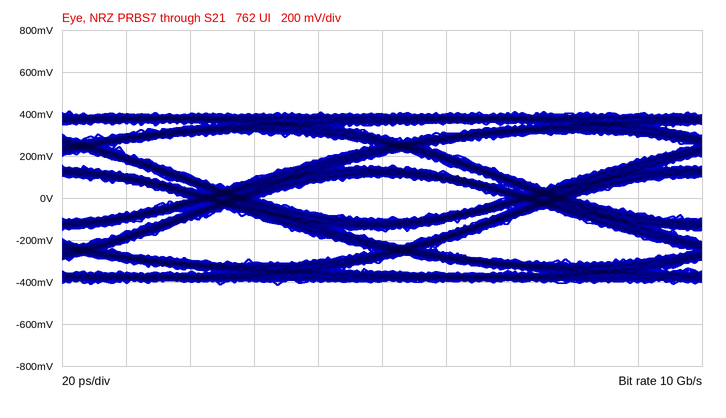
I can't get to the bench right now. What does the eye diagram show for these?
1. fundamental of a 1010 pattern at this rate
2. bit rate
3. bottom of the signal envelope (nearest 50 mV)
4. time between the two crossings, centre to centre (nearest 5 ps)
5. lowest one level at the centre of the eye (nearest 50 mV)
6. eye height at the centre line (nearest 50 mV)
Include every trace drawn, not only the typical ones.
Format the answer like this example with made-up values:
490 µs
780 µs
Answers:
5 GHz
10 Gb/s
-400 mV
100 ps
100 mV
200 mV
